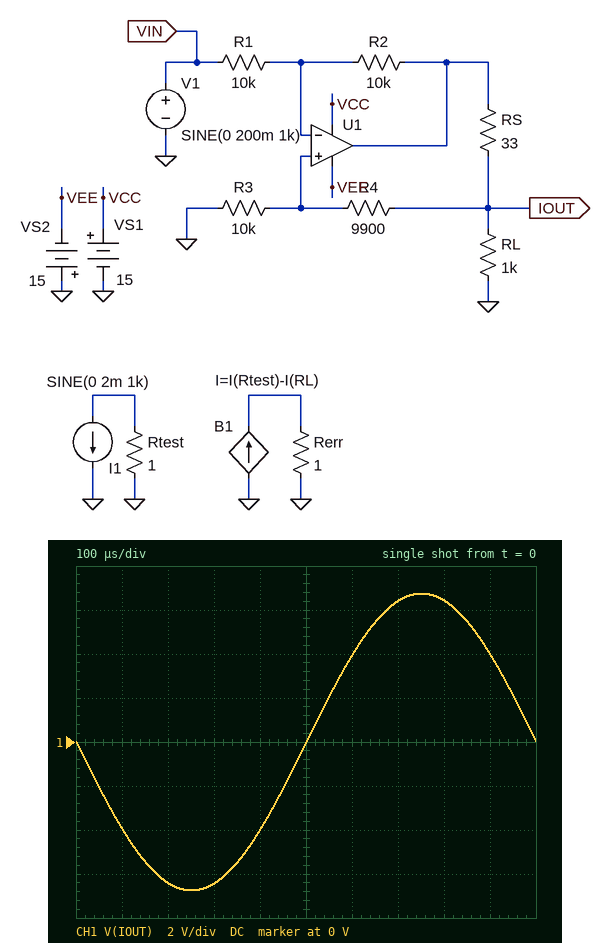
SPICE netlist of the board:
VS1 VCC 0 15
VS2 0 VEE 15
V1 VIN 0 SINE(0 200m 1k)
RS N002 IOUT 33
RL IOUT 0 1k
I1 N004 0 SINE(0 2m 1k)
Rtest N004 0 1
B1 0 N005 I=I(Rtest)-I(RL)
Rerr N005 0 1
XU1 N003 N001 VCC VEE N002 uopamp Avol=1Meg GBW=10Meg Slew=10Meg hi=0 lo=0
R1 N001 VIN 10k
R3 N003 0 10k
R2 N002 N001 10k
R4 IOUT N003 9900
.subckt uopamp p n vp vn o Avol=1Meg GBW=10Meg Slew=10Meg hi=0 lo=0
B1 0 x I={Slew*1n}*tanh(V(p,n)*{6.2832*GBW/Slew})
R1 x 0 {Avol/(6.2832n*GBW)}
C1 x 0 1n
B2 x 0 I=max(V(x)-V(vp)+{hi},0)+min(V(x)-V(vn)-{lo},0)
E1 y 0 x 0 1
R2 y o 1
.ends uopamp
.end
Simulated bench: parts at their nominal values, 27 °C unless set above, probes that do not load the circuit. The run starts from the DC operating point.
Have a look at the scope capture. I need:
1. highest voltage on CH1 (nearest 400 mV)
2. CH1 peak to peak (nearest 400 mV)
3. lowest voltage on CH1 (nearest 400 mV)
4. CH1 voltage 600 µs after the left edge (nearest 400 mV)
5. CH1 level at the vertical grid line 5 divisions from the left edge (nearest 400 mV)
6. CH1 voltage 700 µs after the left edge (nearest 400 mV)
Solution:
6.8 V
13.6 V
-6.8 V
4.0 V
0 V
6.4 V
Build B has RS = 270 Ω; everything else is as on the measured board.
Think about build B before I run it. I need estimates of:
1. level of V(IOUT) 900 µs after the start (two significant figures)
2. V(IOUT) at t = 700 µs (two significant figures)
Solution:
420 mV
680 mV
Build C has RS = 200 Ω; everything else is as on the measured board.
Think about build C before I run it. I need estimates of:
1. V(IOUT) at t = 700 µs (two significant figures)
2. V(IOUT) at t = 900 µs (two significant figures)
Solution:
930 mV
570 mV
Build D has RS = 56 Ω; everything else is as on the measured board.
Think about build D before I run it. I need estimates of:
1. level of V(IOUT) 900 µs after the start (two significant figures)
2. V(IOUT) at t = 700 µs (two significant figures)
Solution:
2.2 V
3.5 V
